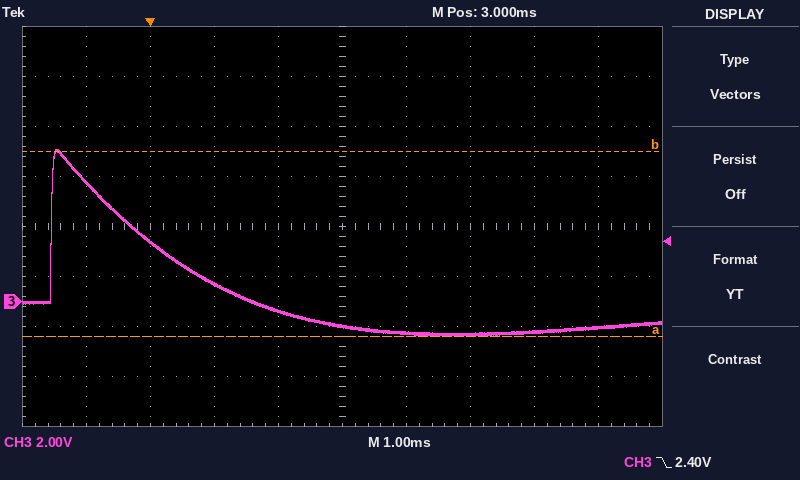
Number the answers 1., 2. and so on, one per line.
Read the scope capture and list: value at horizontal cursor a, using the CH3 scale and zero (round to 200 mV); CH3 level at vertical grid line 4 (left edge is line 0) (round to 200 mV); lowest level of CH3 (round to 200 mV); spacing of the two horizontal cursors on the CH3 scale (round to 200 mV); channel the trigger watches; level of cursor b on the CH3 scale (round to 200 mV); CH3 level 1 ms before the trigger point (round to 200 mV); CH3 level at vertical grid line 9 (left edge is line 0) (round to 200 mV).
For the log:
1. -1.4 V
2. -400 mV
3. -1.4 V
4. 7.4 V
5. CH3
6. 6.0 V
7. 4.8 V
8. -1.0 V
